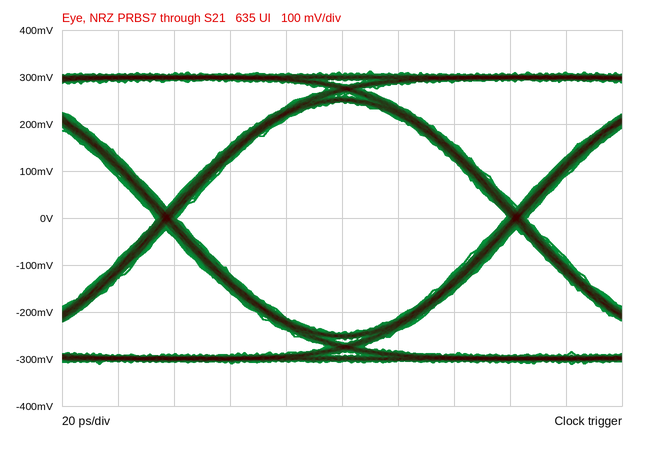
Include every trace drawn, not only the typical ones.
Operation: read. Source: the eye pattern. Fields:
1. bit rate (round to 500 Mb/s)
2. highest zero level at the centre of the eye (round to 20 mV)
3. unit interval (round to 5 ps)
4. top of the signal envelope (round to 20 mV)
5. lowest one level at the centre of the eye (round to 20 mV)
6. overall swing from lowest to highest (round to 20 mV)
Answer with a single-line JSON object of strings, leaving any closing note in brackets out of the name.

{"bit rate": "8.0 Gb/s", "highest zero level at the centre of the eye": "-240 mV", "unit interval": "125 ps", "top of the signal envelope": "320 mV", "lowest one level at the centre of the eye": "240 mV", "overall swing from lowest to highest": "620 mV"}
